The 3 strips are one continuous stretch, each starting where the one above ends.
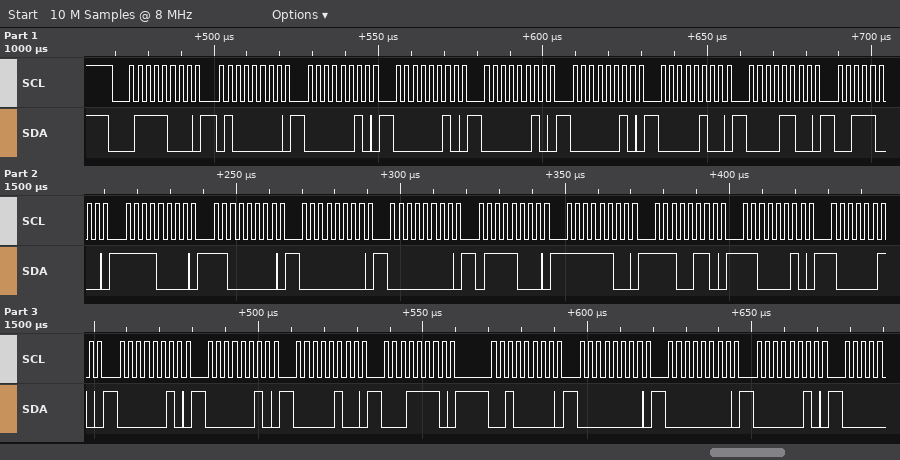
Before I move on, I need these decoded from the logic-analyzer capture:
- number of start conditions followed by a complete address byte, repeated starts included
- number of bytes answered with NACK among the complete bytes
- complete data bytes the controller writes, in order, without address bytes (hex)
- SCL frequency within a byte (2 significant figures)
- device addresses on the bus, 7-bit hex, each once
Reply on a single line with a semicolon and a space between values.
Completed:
1; 0; 40 02 02 02 02 04 0C 38 F0 C0 00 00 78 FC E6 C2 82 02 02 04 1E 20 00 00 02; 400 kHz; 0x3C
